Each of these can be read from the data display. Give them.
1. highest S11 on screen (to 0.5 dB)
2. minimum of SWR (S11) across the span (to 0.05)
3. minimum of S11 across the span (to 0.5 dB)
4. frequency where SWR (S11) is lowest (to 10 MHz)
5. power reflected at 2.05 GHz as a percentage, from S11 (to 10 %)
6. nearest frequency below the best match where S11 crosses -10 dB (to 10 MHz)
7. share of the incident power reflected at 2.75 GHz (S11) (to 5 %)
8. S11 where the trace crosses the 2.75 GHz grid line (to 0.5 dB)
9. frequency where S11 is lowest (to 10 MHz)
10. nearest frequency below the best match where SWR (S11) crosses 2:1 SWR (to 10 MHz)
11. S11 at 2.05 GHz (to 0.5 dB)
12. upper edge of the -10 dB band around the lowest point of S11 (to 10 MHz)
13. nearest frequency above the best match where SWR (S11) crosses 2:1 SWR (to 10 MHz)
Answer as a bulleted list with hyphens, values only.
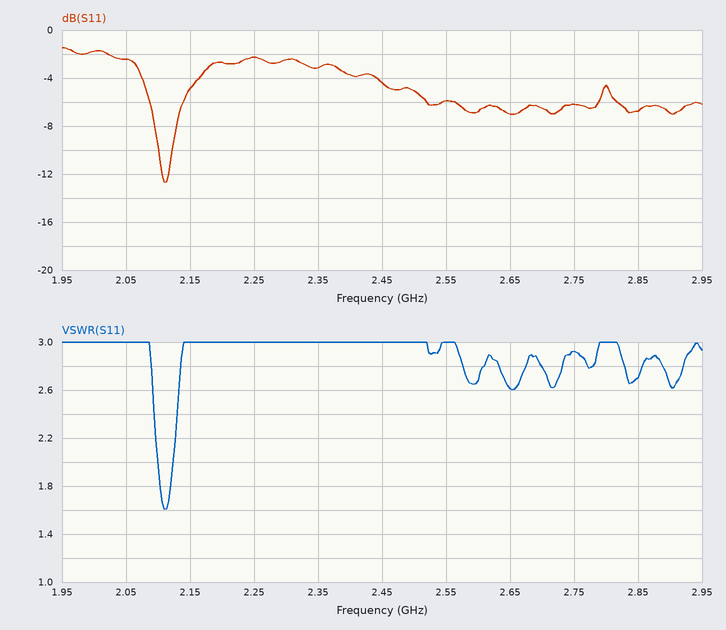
- -1.5 dB
- 1.60
- -12.5 dB
- 2.11 GHz
- 60 %
- 2.10 GHz
- 25 %
- -6.0 dB
- 2.11 GHz
- 2.10 GHz
- -2.5 dB
- 2.12 GHz
- 2.12 GHz
